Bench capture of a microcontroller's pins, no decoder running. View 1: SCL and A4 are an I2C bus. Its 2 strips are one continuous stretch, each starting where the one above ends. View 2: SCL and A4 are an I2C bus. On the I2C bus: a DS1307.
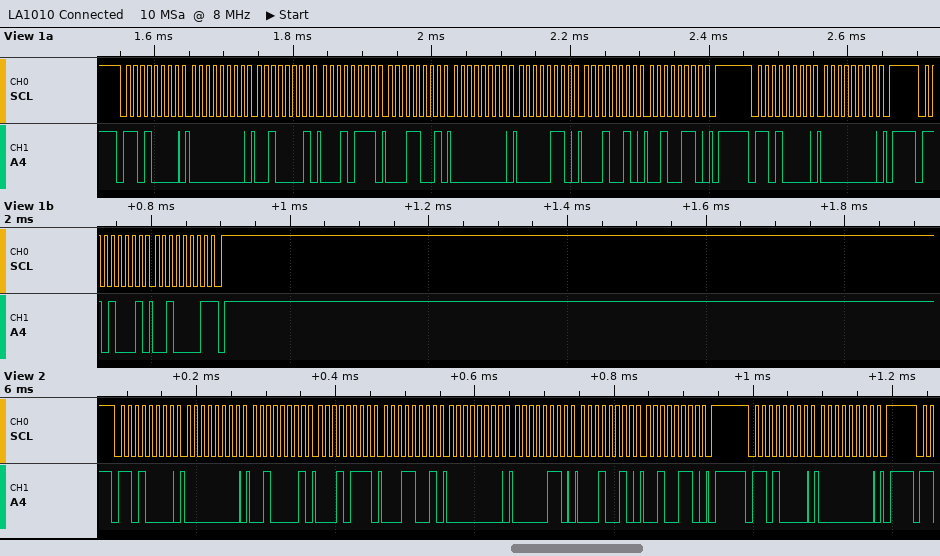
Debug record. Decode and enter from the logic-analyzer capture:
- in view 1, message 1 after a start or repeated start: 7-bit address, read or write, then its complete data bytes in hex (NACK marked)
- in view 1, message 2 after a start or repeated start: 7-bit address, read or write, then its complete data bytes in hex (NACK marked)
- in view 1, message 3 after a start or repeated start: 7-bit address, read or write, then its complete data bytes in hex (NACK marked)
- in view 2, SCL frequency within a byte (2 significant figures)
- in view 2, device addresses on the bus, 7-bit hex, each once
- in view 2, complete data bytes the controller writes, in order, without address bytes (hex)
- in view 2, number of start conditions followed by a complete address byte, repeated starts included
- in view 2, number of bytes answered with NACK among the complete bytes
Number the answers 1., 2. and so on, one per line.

1. 0x68 write: 00 21 17 19 00 06 12 26
2. 0x68 write: 00
3. 0x68 read: 21 NACK
4. 100 kHz
5. 0x68
6. 00 21 17 19 00 06 12 26 00
7. 2
8. 0
